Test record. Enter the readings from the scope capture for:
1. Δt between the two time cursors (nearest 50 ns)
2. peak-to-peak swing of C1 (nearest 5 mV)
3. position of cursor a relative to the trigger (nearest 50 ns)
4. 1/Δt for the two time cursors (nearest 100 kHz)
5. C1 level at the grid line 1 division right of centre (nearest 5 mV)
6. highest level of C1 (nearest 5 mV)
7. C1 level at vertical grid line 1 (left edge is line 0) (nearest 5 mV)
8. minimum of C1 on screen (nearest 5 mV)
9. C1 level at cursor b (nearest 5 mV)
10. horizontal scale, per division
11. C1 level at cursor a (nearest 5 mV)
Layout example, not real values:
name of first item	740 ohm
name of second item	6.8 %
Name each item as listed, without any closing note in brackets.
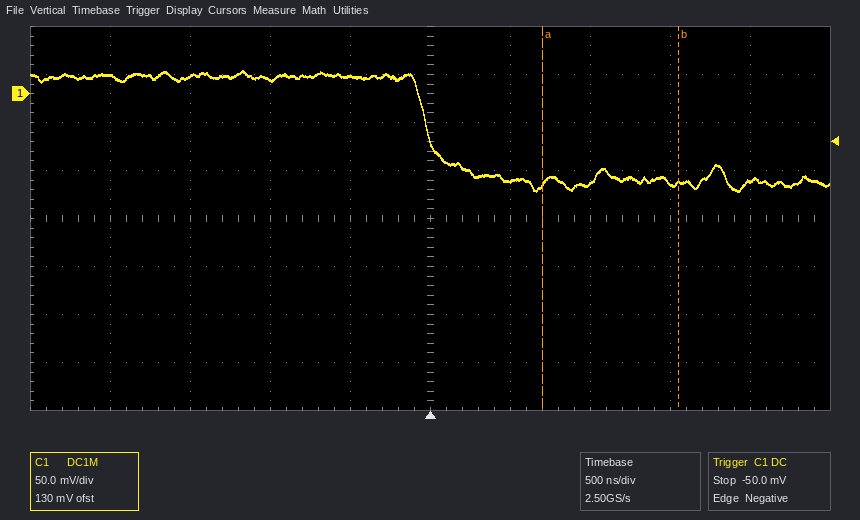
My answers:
Δt between the two time cursors	850 ns
peak-to-peak swing of C1	125 mV
position of cursor a relative to the trigger	+700 ns
1/Δt for the two time cursors	1.2 MHz
C1 level at the grid line 1 division right of centre	-90 mV
highest level of C1	25 mV
C1 level at vertical grid line 1 (left edge is line 0)	20 mV
minimum of C1 on screen	-100 mV
C1 level at cursor b	-95 mV
horizontal scale, per division	500 ns
C1 level at cursor a	-95 mV
